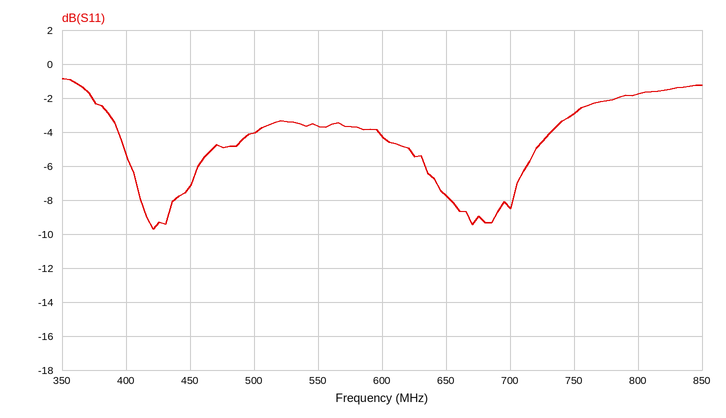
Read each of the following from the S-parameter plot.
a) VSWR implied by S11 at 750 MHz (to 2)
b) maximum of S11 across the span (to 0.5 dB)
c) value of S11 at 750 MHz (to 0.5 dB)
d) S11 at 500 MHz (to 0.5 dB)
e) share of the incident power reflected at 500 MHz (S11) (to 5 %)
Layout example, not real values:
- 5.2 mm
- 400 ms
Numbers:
- 6
- -1.0 dB
- -3.0 dB
- -4.0 dB
- 40 %
